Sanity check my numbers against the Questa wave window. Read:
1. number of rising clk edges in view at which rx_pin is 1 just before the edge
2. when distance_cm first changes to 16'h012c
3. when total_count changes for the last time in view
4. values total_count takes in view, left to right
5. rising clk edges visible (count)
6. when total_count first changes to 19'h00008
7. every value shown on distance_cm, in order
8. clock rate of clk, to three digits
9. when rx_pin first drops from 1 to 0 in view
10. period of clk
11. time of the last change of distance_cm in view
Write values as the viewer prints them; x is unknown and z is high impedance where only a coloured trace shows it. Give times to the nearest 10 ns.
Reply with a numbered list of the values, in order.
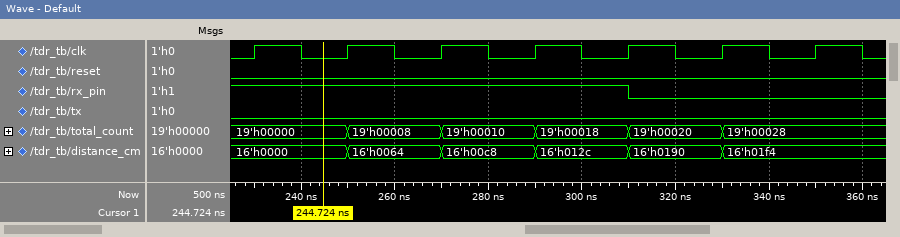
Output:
1. 5
2. 290 ns
3. 330 ns
4. 19'h00000, 19'h00008, 19'h00010, 19'h00018, 19'h00020, 19'h00028
5. 7
6. 250 ns
7. 16'h0000, 16'h0064, 16'h00c8, 16'h012c, 16'h0190, 16'h01f4
8. 50.0 MHz
9. 310 ns
10. 20 ns
11. 330 ns
